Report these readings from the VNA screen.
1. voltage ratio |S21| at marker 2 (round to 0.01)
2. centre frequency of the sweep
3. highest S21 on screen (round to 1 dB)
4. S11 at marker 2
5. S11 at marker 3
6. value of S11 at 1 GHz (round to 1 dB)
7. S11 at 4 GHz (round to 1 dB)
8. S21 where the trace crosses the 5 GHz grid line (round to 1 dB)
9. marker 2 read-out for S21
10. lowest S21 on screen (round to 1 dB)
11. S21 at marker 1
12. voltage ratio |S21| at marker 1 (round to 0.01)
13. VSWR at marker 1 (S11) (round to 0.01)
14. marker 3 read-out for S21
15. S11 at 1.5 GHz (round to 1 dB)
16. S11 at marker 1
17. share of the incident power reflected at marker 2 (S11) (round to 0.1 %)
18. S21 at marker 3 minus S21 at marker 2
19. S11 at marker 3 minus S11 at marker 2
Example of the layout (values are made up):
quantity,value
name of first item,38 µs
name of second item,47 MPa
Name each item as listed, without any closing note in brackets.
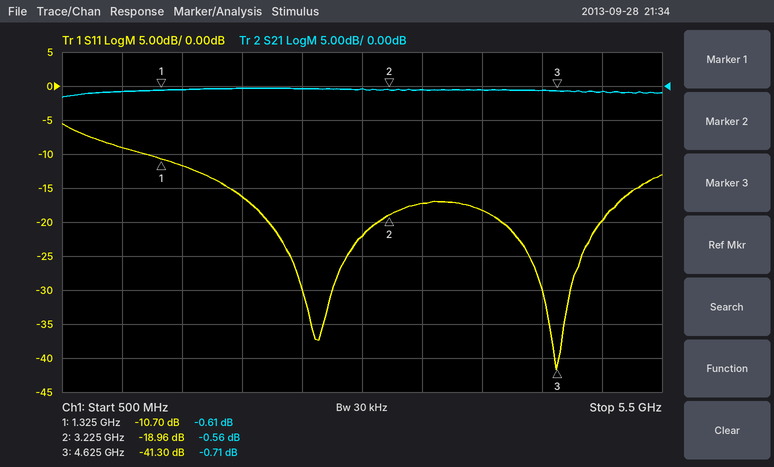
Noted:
quantity,value
voltage ratio |S21| at marker 2,0.94
centre frequency of the sweep,3 GHz
highest S21 on screen,0 dB
S11 at marker 2,-18.96 dB
S11 at marker 3,-41.30 dB
value of S11 at 1 GHz,-9 dB
S11 at 4 GHz,-18 dB
S21 where the trace crosses the 5 GHz grid line,-1 dB
marker 2 read-out for S21,-0.56 dB
lowest S21 on screen,-2 dB
S21 at marker 1,-0.61 dB
voltage ratio |S21| at marker 1,0.93
VSWR at marker 1 (S11),1.82
marker 3 read-out for S21,-0.71 dB
S11 at 1.5 GHz,-12 dB
S11 at marker 1,-10.70 dB
share of the incident power reflected at marker 2 (S11),1.3 %
S21 at marker 3 minus S21 at marker 2,-0.15 dB
S11 at marker 3 minus S11 at marker 2,-22.34 dB
